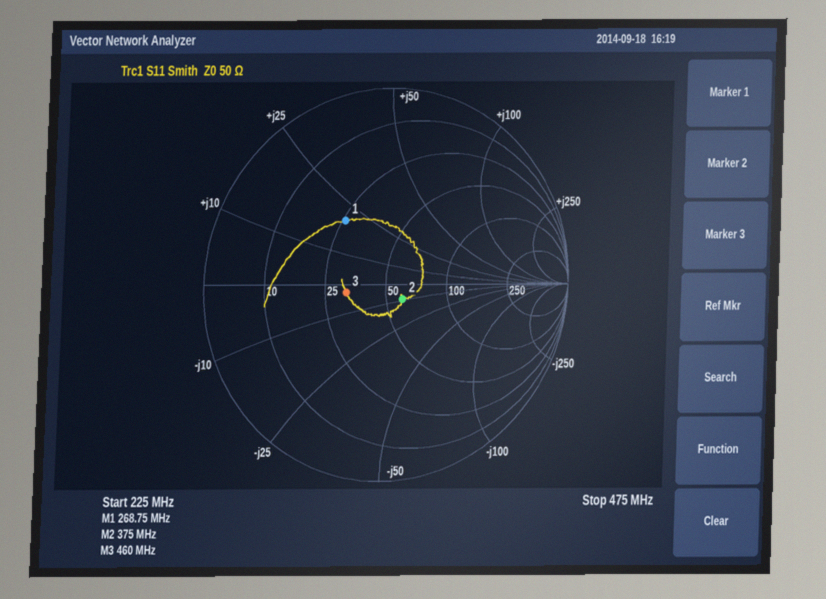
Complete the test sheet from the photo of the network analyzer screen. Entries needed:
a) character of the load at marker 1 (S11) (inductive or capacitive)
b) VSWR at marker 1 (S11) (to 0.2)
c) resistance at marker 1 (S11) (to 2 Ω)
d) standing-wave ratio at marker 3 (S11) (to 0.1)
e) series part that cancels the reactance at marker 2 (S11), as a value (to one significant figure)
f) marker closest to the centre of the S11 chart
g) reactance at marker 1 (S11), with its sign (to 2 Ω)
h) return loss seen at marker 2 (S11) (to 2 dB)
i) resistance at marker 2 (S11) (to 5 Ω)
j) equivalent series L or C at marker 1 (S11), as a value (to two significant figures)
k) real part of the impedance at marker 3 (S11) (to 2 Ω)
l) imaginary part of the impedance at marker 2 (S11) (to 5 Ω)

inductive
2.4
26 Ω
1.6
4 nH
marker 2
+20 Ω
18 dB
60 Ω
12 nH
32 Ω
-10 Ω
